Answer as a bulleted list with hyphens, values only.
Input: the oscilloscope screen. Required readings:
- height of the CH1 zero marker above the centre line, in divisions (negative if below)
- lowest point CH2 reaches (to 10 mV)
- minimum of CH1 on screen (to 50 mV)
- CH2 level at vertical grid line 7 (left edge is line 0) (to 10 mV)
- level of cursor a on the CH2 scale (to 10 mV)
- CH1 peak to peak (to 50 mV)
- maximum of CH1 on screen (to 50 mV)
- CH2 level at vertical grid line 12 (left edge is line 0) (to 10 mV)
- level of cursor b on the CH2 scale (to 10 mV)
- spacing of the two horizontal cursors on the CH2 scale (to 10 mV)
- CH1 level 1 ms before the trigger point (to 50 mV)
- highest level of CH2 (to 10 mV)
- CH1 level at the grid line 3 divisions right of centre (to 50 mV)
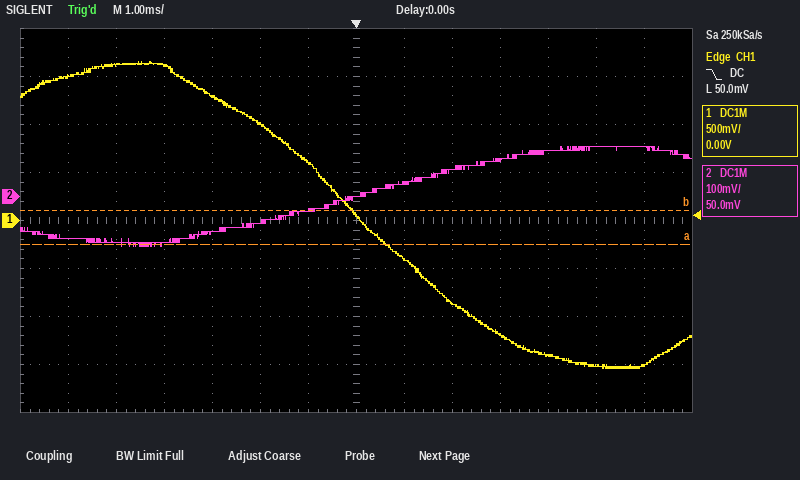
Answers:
- 0.0 div
- -100 mV
- -1.55 V
- 0 mV
- -100 mV
- 3.20 V
- 1.65 V
- 100 mV
- -30 mV
- 70 mV
- 600 mV
- 100 mV
- -1.20 V
